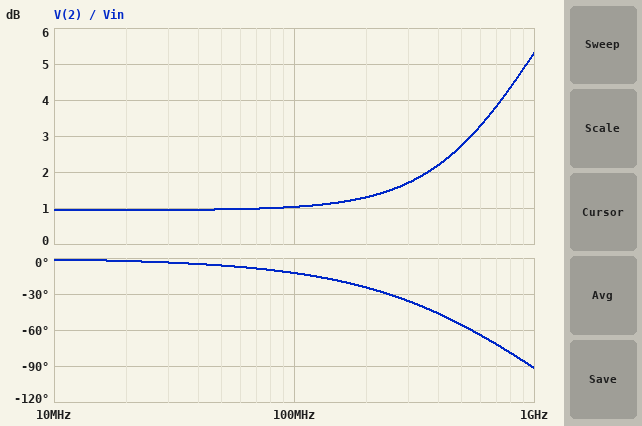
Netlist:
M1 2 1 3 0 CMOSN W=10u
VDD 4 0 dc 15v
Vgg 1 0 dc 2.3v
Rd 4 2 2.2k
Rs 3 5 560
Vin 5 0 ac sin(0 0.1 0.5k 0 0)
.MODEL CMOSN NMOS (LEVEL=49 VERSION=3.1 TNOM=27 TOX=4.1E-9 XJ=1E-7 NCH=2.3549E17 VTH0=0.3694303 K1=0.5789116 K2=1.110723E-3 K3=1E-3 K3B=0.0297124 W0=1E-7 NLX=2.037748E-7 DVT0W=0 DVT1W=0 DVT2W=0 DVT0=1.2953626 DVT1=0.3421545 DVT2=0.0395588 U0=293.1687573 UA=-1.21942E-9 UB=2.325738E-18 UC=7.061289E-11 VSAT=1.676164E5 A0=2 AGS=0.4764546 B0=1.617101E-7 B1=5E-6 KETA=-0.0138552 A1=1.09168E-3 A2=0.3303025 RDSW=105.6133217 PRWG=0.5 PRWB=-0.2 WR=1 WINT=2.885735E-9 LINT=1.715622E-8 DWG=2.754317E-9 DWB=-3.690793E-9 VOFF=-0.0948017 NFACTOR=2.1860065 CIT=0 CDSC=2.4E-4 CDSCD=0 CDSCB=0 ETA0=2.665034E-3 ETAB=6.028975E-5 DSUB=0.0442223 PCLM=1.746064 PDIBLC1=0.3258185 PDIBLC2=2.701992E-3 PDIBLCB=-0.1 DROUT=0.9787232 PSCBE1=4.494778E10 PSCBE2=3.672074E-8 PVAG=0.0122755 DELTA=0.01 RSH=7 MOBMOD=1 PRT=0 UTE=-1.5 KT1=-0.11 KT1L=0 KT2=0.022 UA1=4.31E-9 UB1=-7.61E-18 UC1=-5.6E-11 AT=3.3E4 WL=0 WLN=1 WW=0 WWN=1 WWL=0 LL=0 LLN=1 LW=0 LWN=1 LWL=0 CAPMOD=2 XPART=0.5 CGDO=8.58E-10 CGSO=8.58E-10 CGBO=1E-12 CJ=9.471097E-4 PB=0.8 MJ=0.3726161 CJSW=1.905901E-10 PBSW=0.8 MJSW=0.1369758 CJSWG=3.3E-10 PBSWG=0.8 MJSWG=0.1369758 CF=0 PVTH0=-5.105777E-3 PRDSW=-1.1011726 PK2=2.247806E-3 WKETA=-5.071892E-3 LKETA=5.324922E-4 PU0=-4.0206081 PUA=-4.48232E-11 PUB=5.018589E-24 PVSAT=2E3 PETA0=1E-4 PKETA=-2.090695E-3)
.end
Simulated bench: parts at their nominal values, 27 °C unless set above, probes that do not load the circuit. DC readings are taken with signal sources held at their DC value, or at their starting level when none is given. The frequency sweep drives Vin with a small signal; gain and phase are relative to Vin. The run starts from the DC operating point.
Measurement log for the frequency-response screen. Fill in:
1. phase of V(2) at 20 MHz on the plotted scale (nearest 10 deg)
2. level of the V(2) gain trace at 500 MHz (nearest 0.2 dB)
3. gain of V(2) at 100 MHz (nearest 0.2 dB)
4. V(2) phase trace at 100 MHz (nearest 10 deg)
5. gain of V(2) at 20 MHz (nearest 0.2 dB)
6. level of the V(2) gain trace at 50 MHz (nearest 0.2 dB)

0 deg
2.8 dB
1.0 dB
-10 deg
1.0 dB
1.0 dB
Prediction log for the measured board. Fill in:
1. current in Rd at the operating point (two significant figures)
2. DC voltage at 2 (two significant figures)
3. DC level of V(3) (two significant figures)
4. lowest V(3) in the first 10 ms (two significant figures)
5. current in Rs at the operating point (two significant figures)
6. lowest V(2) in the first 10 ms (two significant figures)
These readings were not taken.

500 µA
14 V
280 mV
210 mV
500 µA
14 V
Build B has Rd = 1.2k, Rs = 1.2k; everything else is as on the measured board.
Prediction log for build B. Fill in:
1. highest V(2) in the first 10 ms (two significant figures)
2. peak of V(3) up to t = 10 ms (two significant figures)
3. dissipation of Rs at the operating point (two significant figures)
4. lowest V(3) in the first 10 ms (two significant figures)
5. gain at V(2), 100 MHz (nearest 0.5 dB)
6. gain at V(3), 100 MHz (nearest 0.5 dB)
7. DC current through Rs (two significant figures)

15 V
510 mV
170 µW
400 mV
-7.5 dB
-5.0 dB
380 µA
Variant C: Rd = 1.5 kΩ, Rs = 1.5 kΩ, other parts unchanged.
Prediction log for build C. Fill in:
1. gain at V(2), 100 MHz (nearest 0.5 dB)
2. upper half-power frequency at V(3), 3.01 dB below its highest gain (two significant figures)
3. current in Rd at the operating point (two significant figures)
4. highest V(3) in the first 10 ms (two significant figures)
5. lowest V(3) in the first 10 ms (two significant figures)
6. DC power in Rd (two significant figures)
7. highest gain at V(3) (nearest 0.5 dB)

-6.5 dB
1.1 GHz
340 µA
570 mV
460 mV
180 µW
-5.5 dB
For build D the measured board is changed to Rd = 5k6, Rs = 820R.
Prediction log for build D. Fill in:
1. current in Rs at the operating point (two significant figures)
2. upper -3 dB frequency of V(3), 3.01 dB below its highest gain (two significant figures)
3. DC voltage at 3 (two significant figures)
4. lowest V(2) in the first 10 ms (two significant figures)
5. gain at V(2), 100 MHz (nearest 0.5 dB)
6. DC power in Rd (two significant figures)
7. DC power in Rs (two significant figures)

440 µA
1.6 GHz
360 mV
12 V
7.5 dB
1.1 mW
160 µW
